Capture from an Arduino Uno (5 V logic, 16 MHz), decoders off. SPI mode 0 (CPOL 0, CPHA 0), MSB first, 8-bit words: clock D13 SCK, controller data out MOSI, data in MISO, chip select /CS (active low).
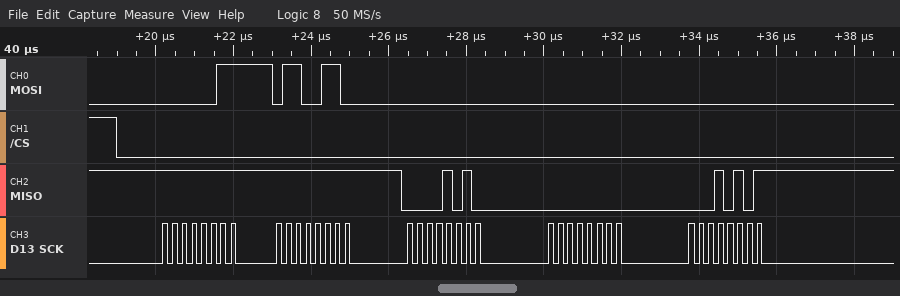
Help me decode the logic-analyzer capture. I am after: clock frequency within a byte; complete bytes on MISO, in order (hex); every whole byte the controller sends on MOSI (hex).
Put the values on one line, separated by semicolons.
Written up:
4 MHz; FF FF 0A 00 15; 03 66 00 00 00
